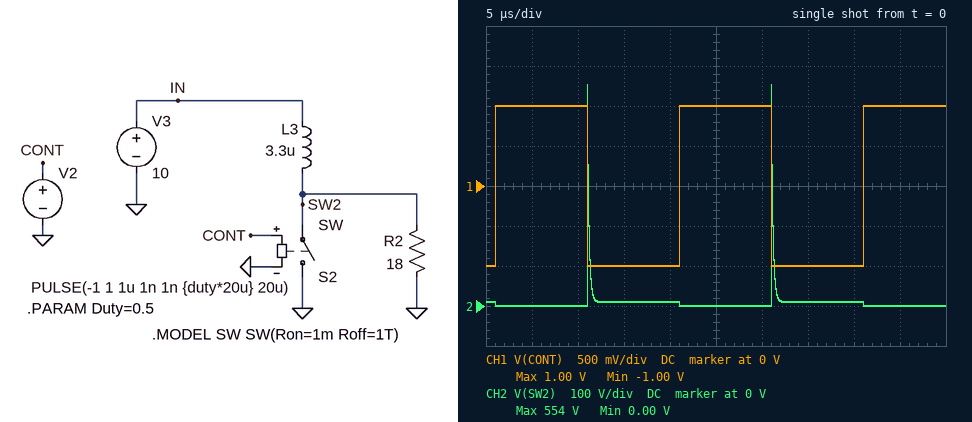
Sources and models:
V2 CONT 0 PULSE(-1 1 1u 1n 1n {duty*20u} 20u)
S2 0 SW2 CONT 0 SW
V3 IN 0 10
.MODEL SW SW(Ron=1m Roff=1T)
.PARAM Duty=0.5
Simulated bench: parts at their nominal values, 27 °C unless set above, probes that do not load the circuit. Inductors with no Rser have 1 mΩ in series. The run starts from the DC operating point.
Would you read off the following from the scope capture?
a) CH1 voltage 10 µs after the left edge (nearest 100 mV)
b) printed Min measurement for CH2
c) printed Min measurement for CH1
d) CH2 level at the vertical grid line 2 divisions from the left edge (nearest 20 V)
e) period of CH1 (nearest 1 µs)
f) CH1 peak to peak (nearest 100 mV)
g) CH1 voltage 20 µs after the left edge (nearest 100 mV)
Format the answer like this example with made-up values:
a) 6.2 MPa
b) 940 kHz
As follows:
a) 1.0 V
b) 0.00 V
c) -1.00 V
d) 0 V
e) 20 µs
f) 2.0 V
g) -1.0 V
